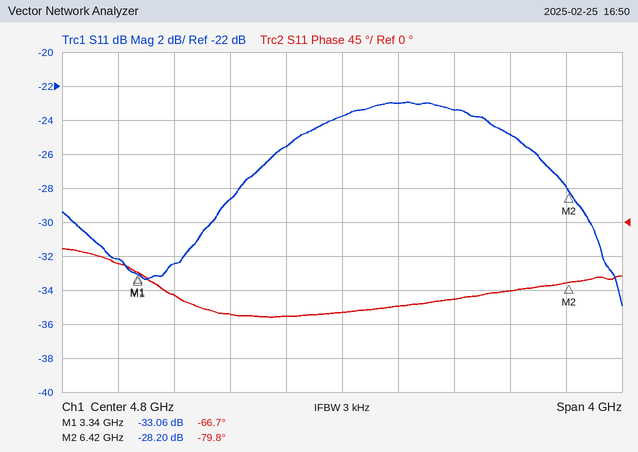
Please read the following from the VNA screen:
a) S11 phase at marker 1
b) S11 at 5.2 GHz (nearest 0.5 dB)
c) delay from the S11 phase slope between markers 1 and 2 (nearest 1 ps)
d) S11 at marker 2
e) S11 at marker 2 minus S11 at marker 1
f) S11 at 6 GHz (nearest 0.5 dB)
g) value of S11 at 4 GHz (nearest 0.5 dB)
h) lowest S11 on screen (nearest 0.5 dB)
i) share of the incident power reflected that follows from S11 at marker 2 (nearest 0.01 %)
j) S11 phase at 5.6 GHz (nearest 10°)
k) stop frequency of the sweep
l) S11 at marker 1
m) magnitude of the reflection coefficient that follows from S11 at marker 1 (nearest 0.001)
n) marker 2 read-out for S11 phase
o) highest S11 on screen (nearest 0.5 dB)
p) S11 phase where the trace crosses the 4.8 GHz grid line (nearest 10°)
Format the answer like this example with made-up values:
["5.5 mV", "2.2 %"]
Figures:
["-66.7°", "-23.0 dB", "12 ps", "-28.20 dB", "4.86 dB", "-25.0 dB", "-28.5 dB", "-35.0 dB", "0.15 %", "-100°", "6.8 GHz", "-33.06 dB", "0.022", "-79.8°", "-23.0 dB", "-120°"]
